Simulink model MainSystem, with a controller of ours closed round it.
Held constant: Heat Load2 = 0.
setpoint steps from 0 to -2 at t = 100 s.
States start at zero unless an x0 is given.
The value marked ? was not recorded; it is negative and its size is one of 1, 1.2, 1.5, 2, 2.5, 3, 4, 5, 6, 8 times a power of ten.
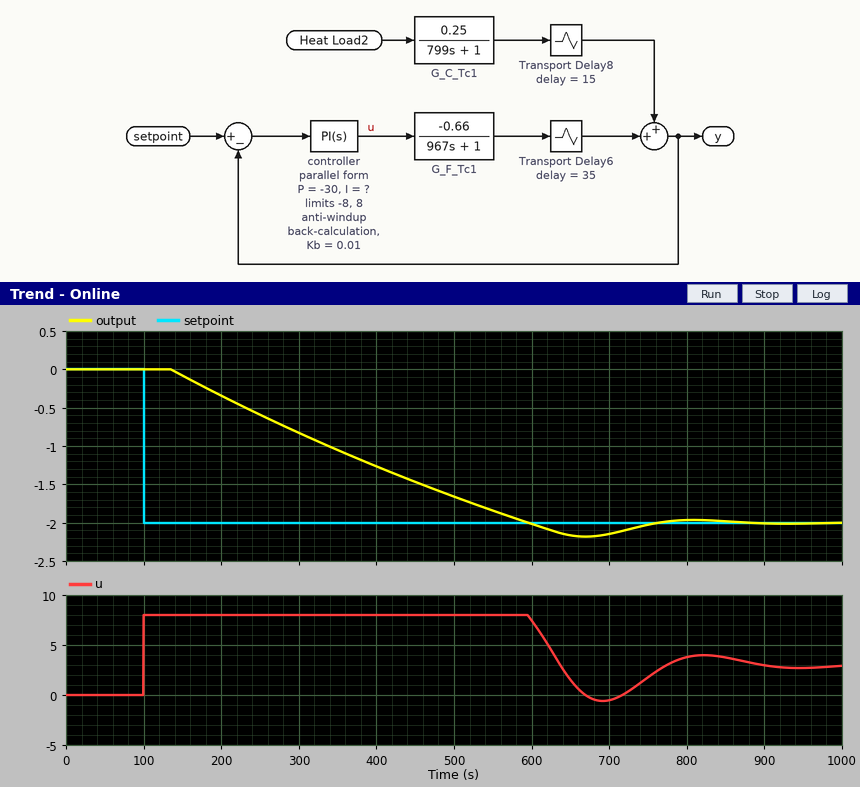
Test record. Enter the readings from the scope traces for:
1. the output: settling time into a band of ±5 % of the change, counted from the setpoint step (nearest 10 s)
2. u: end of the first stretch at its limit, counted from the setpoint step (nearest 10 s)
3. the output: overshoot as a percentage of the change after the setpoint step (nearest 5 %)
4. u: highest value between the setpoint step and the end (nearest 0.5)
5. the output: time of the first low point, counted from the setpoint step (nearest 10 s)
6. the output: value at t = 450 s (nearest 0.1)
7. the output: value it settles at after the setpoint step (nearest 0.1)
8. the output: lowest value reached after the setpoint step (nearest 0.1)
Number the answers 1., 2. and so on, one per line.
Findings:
1. 620 s
2. 500 s
3. 10 %
4. 8.0
5. 570 s
6. -1.5
7. -2.0
8. -2.2
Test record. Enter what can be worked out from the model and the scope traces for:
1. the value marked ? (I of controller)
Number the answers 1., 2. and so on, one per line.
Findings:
1. -0.3
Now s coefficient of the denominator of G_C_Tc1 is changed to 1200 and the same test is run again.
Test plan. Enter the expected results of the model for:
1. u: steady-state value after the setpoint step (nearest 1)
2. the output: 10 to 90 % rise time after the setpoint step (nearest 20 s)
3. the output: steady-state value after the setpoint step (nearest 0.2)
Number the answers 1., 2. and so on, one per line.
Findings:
1. 3
2. 360 s
3. -2.0
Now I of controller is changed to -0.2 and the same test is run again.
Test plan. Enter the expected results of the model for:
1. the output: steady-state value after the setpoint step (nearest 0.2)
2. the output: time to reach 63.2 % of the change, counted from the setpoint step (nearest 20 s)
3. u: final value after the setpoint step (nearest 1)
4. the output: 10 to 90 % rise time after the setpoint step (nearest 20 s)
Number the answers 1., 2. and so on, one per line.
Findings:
1. -2.0
2. 300 s
3. 3
4. 360 s
